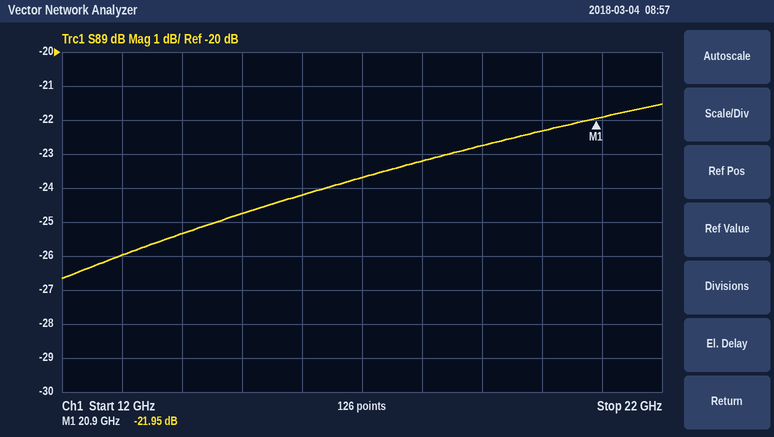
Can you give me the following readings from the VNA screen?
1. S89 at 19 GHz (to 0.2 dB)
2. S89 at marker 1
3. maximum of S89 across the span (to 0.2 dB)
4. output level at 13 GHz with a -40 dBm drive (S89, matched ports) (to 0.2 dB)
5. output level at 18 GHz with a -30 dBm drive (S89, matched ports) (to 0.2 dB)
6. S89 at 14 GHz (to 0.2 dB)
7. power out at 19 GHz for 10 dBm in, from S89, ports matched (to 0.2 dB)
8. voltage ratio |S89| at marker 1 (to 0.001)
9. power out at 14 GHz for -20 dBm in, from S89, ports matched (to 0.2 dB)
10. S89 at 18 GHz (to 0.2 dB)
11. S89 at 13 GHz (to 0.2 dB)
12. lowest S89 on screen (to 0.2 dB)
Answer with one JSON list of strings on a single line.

["-22.8 dB", "-21.95 dB", "-21.6 dB", "-66.0 dBm", "-53.2 dBm", "-25.4 dB", "-12.8 dBm", "0.080", "-45.4 dBm", "-23.2 dB", "-26.0 dB", "-26.6 dB"]
